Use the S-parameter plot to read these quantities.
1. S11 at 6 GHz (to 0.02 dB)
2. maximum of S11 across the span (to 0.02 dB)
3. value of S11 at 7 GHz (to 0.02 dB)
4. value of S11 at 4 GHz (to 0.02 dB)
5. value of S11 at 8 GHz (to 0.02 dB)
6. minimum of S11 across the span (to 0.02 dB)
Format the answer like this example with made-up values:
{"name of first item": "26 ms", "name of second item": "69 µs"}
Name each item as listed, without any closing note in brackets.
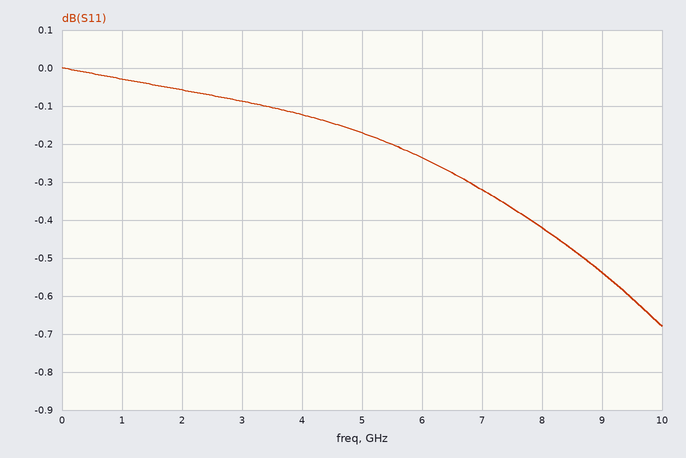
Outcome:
{"S11 at 6 GHz": "-0.24 dB", "maximum of S11 across the span": "0.00 dB", "value of S11 at 7 GHz": "-0.32 dB", "value of S11 at 4 GHz": "-0.12 dB", "value of S11 at 8 GHz": "-0.42 dB", "minimum of S11 across the span": "-0.68 dB"}
